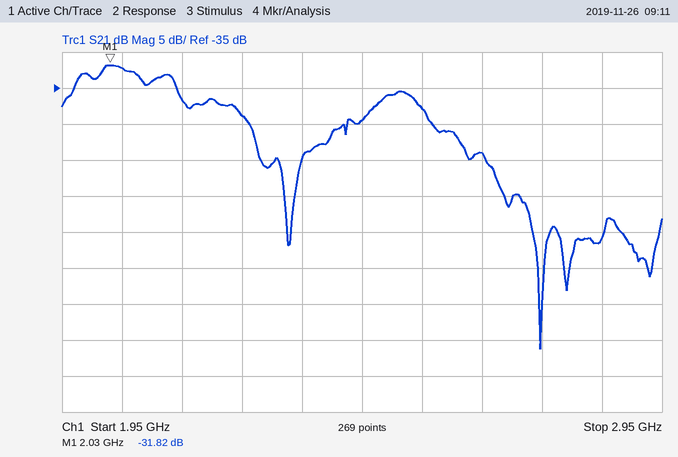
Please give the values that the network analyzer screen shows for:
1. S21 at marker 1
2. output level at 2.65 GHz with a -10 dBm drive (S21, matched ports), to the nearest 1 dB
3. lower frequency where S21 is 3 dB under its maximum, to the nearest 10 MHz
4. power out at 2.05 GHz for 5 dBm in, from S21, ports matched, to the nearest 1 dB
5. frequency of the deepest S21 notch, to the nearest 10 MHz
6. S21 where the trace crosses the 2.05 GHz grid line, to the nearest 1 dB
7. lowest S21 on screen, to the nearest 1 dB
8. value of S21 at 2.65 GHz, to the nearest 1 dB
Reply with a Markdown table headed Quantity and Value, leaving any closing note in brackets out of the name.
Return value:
| Quantity | Value |
|---|---|
| S21 at marker 1 | -31.82 dB |
| output level at 2.65 GHz with a -10 dBm drive (S21, matched ports), to the nearest 1 dB | -54 dBm |
| lower frequency where S21 is 3 dB under its maximum, to the nearest 10 MHz | 1.97 GHz |
| power out at 2.05 GHz for 5 dBm in, from S21, ports matched, to the nearest 1 dB | -27 dBm |
| frequency of the deepest S21 notch, to the nearest 10 MHz | 2.75 GHz |
| S21 where the trace crosses the 2.05 GHz grid line, to the nearest 1 dB | -32 dB |
| lowest S21 on screen, to the nearest 1 dB | -71 dB |
| value of S21 at 2.65 GHz, to the nearest 1 dB | -44 dB |
